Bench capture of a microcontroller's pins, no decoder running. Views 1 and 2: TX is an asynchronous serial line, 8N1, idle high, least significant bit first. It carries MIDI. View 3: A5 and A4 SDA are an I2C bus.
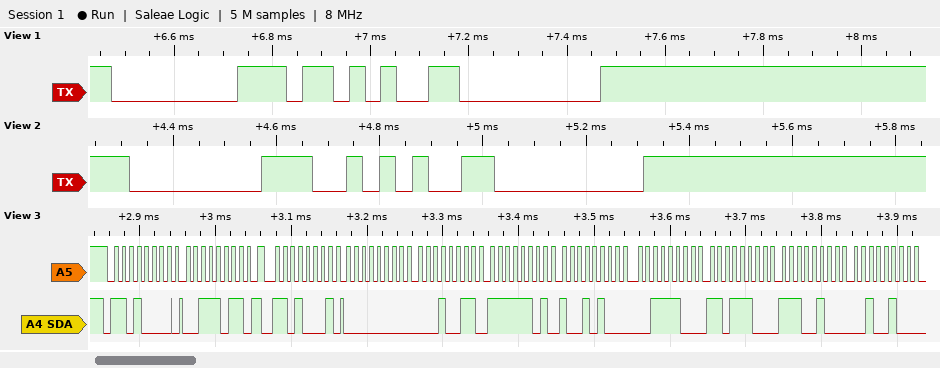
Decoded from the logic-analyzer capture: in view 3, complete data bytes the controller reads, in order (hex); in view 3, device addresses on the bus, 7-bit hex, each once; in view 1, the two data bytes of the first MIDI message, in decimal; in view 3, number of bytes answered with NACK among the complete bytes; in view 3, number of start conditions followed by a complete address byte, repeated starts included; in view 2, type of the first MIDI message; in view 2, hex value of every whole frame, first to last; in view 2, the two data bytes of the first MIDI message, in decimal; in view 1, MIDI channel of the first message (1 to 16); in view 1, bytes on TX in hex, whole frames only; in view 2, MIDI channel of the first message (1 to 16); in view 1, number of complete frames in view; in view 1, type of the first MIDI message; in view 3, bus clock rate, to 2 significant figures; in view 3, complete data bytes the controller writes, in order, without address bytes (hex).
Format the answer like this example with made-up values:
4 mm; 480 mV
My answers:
00 13 FD 94 3C DC E4 24; 0x68; 43, 0; 0; 2; Note Off; 0x80 0x2A 0x00; 42, 0; 1; 80 2B 00; 1; 3; Note Off; 100 kHz; 3B
